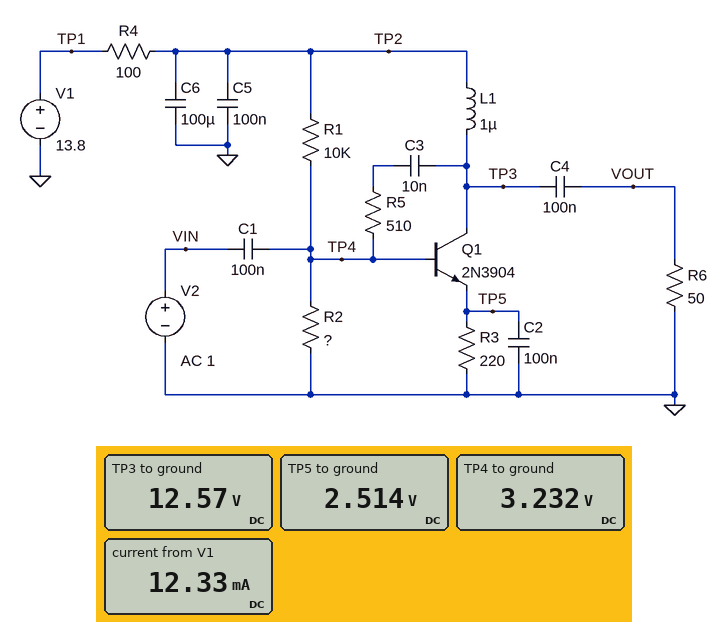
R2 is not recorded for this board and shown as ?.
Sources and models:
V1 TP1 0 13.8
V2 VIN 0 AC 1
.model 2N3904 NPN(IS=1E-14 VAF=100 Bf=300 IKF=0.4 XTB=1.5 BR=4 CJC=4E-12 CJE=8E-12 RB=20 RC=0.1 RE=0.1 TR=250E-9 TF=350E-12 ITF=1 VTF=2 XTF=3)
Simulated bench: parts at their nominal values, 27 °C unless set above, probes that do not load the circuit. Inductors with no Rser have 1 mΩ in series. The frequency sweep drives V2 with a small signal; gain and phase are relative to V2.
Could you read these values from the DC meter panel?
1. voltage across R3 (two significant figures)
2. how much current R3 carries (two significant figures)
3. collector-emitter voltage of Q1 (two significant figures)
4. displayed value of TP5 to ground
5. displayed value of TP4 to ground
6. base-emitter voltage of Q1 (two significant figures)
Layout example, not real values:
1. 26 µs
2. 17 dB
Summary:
1. 2.5 V
2. 11 mA
3. 10 V
4. 2.514 V
5. 3.232 V
6. 720 mV
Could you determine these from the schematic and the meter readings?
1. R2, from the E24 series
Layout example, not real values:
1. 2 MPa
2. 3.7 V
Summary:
1. 3.6 kΩ
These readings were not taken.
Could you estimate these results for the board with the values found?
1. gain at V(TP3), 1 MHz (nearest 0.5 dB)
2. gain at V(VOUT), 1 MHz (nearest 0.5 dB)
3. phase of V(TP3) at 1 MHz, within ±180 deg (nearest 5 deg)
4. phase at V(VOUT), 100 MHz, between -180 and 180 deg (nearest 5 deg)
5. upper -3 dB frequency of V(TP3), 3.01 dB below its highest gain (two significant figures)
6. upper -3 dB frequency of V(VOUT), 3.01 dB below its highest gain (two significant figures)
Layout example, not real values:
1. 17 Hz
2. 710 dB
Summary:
1. 6.5 dB
2. 6.5 dB
3. -65 deg
4. 115 deg
5. 54 MHz
6. 54 MHz
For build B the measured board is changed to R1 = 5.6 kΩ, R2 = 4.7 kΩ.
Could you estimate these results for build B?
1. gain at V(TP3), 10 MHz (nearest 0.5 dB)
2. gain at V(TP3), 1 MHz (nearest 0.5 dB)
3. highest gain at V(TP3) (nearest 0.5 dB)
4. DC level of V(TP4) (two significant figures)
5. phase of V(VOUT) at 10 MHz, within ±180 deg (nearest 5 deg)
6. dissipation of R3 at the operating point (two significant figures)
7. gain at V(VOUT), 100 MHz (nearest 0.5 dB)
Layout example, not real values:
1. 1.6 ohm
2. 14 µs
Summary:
1. 27.5 dB
2. 9.0 dB
3. 28.0 dB
4. 5.2 V
5. -160 deg
6. 89 mW
7. 17.5 dB
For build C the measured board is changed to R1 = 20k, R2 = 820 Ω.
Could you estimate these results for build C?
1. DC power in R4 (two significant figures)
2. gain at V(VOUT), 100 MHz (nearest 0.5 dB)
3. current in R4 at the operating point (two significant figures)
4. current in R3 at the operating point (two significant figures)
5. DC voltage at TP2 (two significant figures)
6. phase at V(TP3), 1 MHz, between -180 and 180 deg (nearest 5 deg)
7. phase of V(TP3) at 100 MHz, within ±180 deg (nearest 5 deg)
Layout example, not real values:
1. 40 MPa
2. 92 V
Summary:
1. 45 µW
2. -21.0 dB
3. 670 µA
4. 12 µA
5. 14 V
6. 85 deg
7. 35 deg
